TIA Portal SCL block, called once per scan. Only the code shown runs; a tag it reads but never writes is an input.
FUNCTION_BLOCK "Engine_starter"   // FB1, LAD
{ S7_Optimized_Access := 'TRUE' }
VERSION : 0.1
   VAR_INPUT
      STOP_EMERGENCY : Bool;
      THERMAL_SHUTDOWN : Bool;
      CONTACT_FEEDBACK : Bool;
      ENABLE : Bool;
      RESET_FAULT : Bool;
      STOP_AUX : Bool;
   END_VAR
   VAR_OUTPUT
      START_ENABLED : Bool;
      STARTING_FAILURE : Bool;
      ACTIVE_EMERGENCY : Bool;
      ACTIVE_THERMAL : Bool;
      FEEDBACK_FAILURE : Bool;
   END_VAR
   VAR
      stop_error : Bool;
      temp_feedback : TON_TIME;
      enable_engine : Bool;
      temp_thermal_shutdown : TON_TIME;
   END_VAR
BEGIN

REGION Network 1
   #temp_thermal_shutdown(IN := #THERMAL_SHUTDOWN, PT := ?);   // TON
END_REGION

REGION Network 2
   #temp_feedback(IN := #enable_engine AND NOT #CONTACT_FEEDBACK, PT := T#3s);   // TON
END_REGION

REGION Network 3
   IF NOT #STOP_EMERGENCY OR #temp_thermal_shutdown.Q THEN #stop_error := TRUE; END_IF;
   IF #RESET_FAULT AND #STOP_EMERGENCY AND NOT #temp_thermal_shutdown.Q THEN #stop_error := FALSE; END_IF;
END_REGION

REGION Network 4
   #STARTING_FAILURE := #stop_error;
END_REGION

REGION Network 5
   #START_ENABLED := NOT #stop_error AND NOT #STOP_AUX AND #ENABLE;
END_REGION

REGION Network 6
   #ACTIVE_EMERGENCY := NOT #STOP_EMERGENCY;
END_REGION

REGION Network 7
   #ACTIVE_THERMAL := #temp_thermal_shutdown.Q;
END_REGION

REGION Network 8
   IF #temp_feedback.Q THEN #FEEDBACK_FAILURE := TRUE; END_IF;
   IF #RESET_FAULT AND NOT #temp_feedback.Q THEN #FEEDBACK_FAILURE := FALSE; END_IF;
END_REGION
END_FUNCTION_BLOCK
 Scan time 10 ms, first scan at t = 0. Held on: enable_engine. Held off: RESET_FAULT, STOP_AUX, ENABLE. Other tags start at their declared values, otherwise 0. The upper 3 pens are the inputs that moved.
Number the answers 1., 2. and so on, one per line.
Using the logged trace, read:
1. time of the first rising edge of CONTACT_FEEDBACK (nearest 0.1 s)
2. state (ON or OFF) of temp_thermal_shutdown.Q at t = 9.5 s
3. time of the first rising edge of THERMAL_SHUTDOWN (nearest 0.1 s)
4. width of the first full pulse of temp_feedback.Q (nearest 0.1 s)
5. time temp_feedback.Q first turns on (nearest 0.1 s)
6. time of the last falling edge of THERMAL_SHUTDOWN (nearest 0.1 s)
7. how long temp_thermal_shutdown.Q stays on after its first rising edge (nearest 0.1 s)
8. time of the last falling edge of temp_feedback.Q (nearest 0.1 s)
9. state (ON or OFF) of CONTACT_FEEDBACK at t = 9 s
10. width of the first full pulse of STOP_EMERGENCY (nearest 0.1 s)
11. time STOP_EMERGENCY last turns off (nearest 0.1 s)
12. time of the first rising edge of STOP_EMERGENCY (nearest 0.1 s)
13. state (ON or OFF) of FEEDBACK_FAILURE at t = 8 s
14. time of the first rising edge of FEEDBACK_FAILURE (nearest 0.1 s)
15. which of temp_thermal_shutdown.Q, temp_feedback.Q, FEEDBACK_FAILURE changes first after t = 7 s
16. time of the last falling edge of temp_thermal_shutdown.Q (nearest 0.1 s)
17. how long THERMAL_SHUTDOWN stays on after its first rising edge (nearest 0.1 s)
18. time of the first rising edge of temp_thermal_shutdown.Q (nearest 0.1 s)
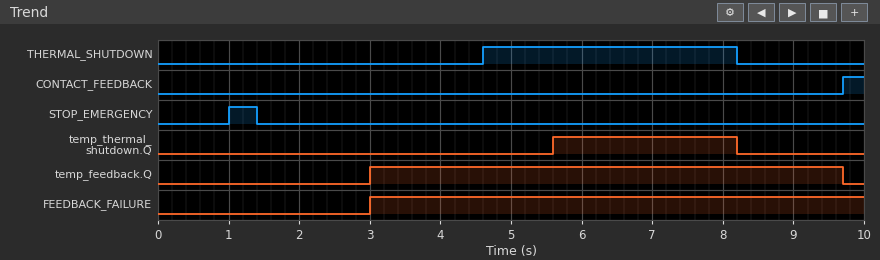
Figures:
1. 9.7 s
2. OFF
3. 4.6 s
4. 6.7 s
5. 3.0 s
6. 8.2 s
7. 2.6 s
8. 9.7 s
9. OFF
10. 0.4 s
11. 1.4 s
12. 1.0 s
13. ON
14. 3.0 s
15. temp_thermal_shutdown.Q
16. 8.2 s
17. 3.6 s
18. 5.6 s
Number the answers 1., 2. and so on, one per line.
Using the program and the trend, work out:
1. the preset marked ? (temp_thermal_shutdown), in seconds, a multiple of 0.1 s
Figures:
1. 1.0 s
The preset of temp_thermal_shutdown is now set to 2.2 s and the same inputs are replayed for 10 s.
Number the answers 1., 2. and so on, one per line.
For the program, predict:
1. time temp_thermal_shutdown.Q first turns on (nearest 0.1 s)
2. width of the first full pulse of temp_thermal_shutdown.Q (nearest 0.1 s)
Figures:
1. 6.8 s
2. 1.4 s
